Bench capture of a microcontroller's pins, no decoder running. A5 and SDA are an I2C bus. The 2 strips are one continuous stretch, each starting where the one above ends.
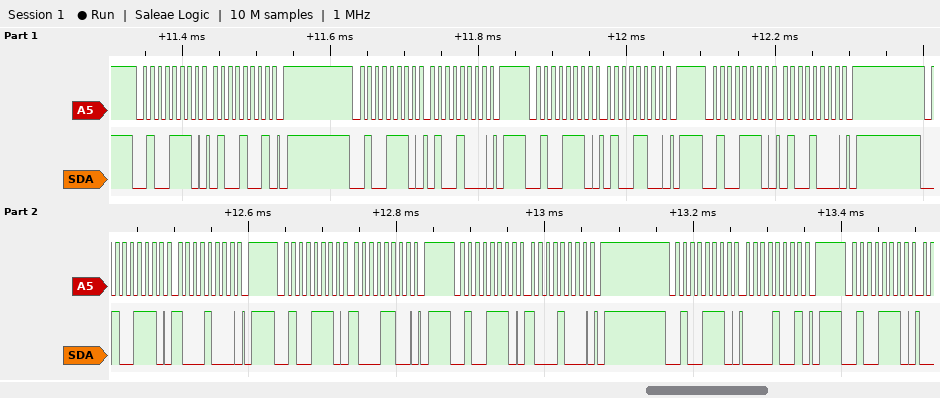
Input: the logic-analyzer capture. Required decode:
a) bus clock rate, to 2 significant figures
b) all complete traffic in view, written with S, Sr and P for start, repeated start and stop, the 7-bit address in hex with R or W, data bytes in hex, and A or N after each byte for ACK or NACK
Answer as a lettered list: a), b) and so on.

a) 100 kHz
b) S 27W A 49 A P S 27W A 48 A P S 27W A 4C A P S 27W A 48 A P S 27W A 88 A P S 27W A 8C A P S 27W A 88 A P S 27W A 09 A P S 27W A
